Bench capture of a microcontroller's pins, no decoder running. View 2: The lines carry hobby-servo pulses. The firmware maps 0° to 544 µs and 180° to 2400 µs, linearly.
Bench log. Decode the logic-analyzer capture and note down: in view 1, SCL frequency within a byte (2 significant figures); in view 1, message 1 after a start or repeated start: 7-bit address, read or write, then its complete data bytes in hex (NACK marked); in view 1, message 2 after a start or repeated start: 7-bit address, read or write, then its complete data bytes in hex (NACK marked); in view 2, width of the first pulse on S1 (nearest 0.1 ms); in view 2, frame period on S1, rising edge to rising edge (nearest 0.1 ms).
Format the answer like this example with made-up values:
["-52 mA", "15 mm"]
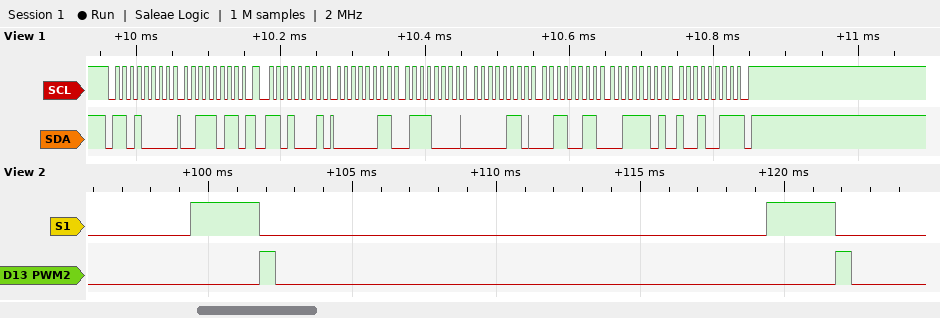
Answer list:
["100 kHz", "0x68 write: 3B", "0x68 read: 03 70 06 33 3D 93 NACK", "2.4 ms", "20.0 ms"]
